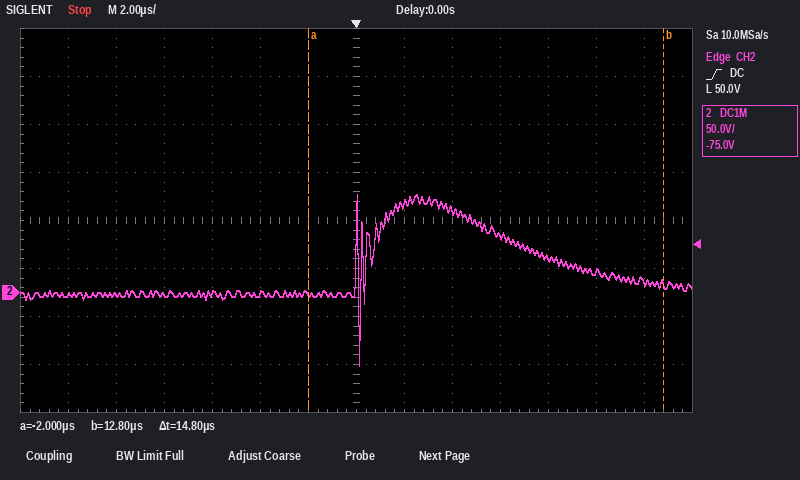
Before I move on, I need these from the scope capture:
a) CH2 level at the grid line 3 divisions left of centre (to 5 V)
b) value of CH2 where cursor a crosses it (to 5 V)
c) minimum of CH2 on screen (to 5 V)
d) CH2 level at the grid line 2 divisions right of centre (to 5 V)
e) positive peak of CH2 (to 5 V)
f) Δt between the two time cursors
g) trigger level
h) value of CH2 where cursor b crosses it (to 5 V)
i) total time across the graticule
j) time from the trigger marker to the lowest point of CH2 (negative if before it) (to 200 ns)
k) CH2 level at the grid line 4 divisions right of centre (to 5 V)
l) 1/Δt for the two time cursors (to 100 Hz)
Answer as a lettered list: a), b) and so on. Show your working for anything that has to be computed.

a) 0 V
b) 0 V
c) -75 V
d) 85 V
e) 100 V
f) 14.8 µs
g) 50.0 V
h) 10 V
i) 28 µs
j) +200 ns
k) 35 V
l) 1 / 14.8 µs ≈ 67.6 kHz
